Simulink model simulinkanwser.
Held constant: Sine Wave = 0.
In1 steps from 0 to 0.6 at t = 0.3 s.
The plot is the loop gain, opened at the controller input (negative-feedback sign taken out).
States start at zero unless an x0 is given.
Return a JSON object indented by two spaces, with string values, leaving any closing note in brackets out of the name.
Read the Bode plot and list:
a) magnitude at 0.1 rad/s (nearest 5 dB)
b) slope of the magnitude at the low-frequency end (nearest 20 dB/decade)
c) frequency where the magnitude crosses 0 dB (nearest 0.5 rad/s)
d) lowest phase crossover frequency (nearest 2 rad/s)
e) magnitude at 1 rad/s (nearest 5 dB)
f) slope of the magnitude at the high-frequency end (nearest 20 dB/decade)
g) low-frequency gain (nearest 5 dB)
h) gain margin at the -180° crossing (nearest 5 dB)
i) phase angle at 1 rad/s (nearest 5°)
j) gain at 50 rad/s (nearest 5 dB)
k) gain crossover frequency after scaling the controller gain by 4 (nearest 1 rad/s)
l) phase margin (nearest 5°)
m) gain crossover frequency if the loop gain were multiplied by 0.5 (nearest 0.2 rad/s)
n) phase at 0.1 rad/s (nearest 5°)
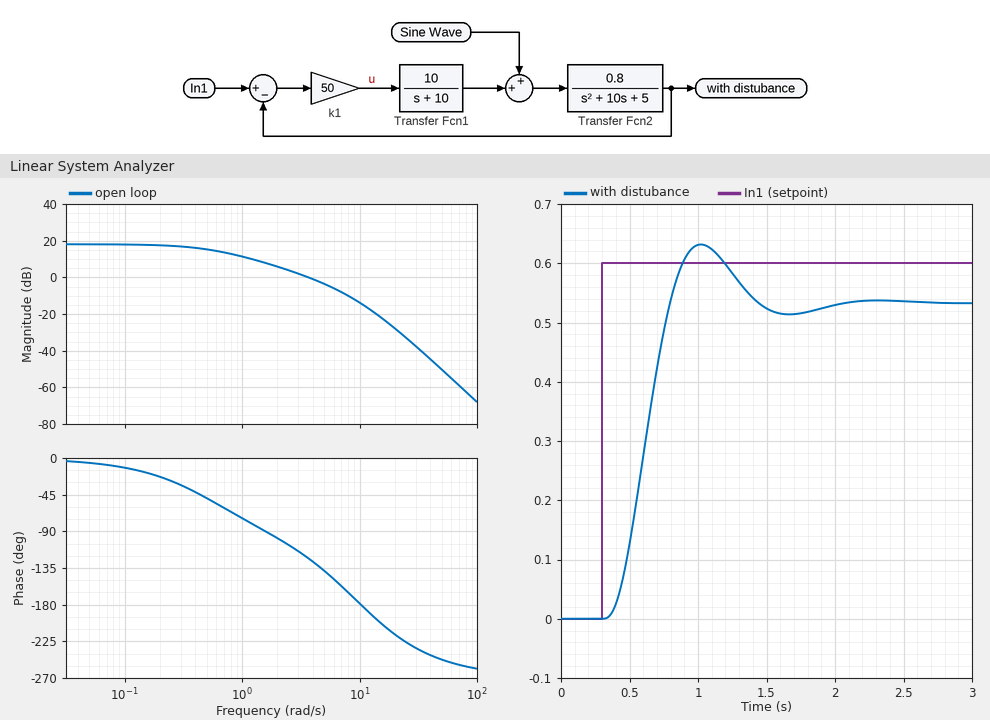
{
  "magnitude at 0.1 rad/s": "20 dB",
  "slope of the magnitude at the low-frequency end": "0 dB/decade",
  "frequency where the magnitude crosses 0 dB": "3.5 rad/s",
  "lowest phase crossover frequency": "10 rad/s",
  "magnitude at 1 rad/s": "10 dB",
  "slope of the magnitude at the high-frequency end": "-60 dB/decade",
  "low-frequency gain": "20 dB",
  "gain margin at the -180° crossing": "15 dB",
  "phase angle at 1 rad/s": "-75°",
  "gain at 50 rad/s": "-50 dB",
  "gain crossover frequency after scaling the controller gain by 4": "9 rad/s",
  "phase margin": "55°",
  "gain crossover frequency if the loop gain were multiplied by 0.5": "2.0 rad/s",
  "phase at 0.1 rad/s": "-10°"
}
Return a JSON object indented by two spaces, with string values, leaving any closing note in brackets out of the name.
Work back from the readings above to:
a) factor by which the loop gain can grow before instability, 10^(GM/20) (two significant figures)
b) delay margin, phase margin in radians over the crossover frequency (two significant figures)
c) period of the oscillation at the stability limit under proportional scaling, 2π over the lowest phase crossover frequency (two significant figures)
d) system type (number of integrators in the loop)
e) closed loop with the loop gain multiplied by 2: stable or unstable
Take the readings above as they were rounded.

{
  "factor by which the loop gain can grow before instability, 10^(GM/20)": "5.6",
  "delay margin, phase margin in radians over the crossover frequency": "0.27 s",
  "period of the oscillation at the stability limit under proportional scaling, 2π over the lowest phase crossover frequency": "0.63 s",
  "system type": "0",
  "closed loop with the loop gain multiplied by 2: stable or unstable": "stable"
}
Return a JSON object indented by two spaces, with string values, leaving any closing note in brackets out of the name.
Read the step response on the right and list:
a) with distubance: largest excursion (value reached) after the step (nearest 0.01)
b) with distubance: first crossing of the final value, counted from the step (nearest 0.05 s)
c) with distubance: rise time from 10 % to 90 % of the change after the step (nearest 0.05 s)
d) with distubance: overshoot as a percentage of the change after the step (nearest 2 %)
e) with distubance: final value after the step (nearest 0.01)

{
  "with distubance: largest excursion (value reached) after the step": "0.63",
  "with distubance: first crossing of the final value, counted from the step": "0.50 s",
  "with distubance: rise time from 10 % to 90 % of the change after the step": "0.30 s",
  "with distubance: overshoot as a percentage of the change after the step": "18 %",
  "with distubance: final value after the step": "0.53"
}
